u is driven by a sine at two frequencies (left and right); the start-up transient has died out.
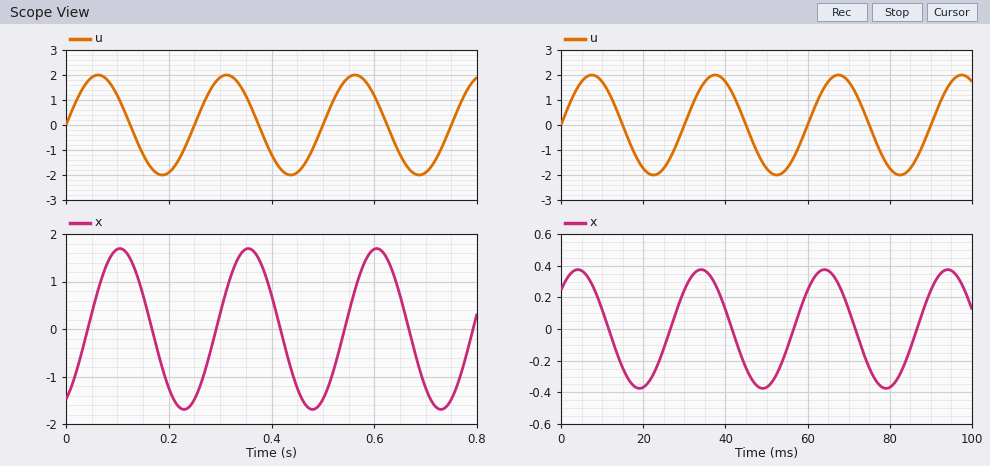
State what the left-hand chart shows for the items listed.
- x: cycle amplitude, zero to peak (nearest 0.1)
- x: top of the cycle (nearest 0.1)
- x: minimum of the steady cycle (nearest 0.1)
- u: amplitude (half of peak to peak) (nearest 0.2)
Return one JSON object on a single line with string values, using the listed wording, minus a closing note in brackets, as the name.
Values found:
{"x: cycle amplitude, zero to peak": "1.7", "x: top of the cycle": "1.7", "x: minimum of the steady cycle": "-1.7", "u: amplitude (half of peak to peak)": "2.0"}
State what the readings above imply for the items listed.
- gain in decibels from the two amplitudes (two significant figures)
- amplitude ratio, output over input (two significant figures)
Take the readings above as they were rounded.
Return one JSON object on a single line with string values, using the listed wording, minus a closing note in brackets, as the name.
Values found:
{"gain in decibels from the two amplitudes": "-1.4 dB", "amplitude ratio, output over input": "0.85"}
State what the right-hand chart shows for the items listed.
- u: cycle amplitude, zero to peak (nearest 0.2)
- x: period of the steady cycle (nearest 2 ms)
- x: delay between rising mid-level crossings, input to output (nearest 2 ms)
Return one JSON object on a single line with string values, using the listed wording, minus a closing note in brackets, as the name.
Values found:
{"u: cycle amplitude, zero to peak": "2.0", "x: period of the steady cycle": "30 ms", "x: delay between rising mid-level crossings, input to output": "26 ms"}
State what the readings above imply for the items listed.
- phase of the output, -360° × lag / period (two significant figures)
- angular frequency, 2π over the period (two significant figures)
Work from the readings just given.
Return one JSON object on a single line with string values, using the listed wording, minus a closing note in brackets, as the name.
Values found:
{"phase of the output, -360° × lag / period": "-310°", "angular frequency, 2π over the period": "0.21 rad/ms"}
